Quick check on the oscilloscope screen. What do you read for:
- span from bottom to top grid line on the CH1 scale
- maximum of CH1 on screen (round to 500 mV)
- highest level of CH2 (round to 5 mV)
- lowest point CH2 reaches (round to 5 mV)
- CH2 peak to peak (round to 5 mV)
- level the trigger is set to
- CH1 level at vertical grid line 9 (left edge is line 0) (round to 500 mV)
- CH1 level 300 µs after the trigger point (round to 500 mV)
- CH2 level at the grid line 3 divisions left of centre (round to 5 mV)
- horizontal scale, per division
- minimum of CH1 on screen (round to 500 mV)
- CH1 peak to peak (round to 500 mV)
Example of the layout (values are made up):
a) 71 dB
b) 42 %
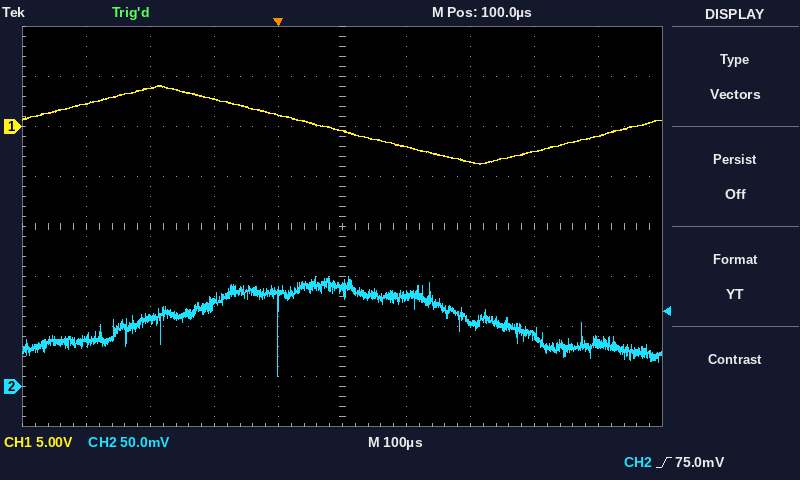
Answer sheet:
a) 40 V
b) 4.0 V
c) 110 mV
d) 10 mV
e) 100 mV
f) 75.0 mV
g) -1.0 V
h) -3.5 V
i) 65 mV
j) 100 µs
k) -4.0 V
l) 8.0 V
